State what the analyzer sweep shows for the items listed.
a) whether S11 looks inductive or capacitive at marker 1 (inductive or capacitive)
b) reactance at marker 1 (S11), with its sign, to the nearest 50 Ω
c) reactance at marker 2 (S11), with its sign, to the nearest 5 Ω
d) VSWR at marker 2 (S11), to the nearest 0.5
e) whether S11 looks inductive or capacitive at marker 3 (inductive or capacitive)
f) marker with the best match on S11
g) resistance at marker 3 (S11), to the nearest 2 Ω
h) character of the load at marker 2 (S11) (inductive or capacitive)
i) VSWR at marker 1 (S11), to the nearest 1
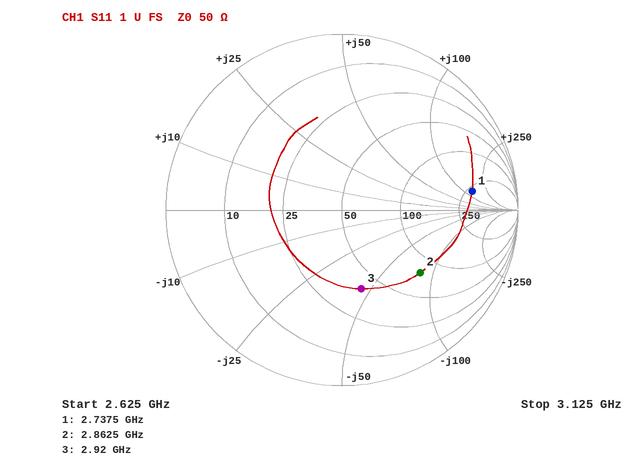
inductive
+150 Ω
-80 Ω
3.5
capacitive
marker 3
40 Ω
capacitive
7
